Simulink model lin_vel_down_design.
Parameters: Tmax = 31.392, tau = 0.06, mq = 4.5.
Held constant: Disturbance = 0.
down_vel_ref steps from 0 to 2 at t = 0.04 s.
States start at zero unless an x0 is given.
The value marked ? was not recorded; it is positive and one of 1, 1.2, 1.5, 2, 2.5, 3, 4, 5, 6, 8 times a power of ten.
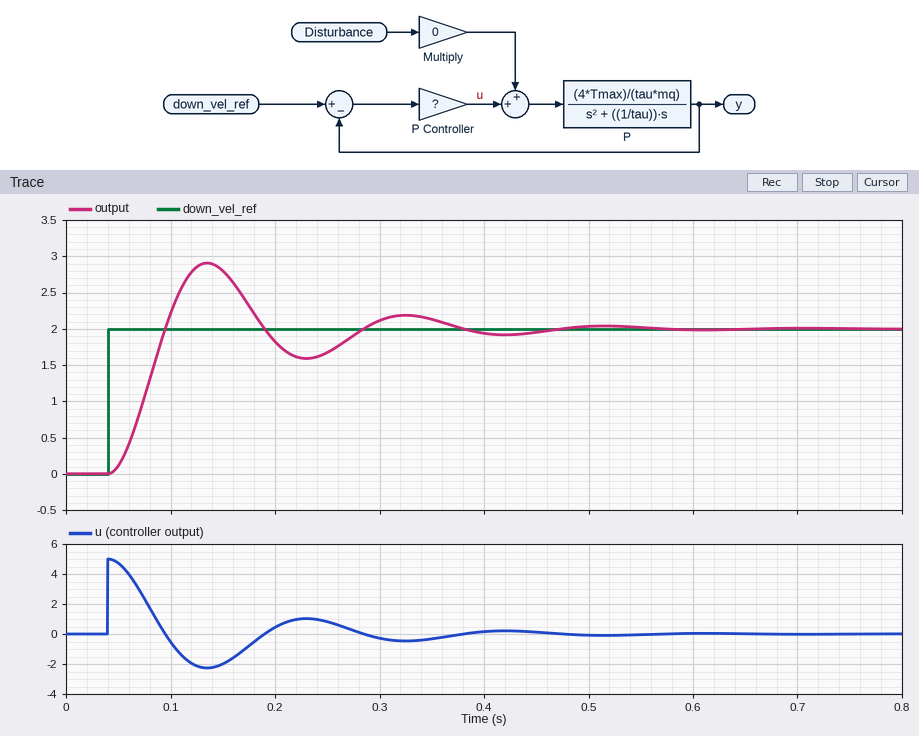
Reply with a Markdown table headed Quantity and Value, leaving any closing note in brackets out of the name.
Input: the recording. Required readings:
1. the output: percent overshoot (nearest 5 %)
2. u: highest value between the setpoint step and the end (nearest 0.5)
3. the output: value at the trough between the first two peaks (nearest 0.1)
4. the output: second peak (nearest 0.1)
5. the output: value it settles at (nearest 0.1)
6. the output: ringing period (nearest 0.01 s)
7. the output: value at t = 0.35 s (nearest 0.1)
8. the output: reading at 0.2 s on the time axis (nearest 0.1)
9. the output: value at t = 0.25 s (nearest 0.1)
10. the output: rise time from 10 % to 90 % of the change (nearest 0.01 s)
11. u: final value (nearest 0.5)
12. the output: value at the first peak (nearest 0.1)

| Quantity | Value |
|---|---|
| the output: percent overshoot | 45 % |
| u: highest value between the setpoint step and the end | 5.0 |
| the output: value at the trough between the first two peaks | 1.6 |
| the output: second peak | 2.2 |
| the output: value it settles at | 2.0 |
| the output: ringing period | 0.19 s |
| the output: value at t = 0.35 s | 2.1 |
| the output: reading at 0.2 s on the time axis | 1.8 |
| the output: value at t = 0.25 s | 1.7 |
| the output: rise time from 10 % to 90 % of the change | 0.04 s |
| u: final value | 0.0 |
| the output: value at the first peak | 2.9 |
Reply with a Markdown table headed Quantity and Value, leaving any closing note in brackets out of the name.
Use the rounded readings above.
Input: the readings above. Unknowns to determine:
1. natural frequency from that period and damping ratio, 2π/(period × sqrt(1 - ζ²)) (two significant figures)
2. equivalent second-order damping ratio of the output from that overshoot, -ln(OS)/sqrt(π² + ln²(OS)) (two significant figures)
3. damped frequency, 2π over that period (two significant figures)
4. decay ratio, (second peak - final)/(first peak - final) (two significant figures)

| Quantity | Value |
|---|---|
| natural frequency from that period and damping ratio, 2π/(period × sqrt(1 - ζ²)) | 34 rad/s |
| equivalent second-order damping ratio of the output from that overshoot, -ln(OS)/sqrt(π² + ln²(OS)) | 0.25 |
| damped frequency, 2π over that period | 33 rad/s |
| decay ratio, (second peak - final)/(first peak - final) | 0.22 |
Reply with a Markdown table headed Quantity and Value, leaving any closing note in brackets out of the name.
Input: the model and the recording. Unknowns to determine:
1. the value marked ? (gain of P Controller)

| Quantity | Value |
|---|---|
| the value marked ? | 2.5 |
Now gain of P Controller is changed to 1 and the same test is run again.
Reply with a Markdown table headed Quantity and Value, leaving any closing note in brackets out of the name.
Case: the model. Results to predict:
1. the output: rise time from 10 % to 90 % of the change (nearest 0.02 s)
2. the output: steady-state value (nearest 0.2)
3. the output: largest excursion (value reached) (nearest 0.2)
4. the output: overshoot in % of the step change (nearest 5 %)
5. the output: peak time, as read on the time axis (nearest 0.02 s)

| Quantity | Value |
|---|---|
| the output: rise time from 10 % to 90 % of the change | 0.06 s |
| the output: steady-state value | 2.0 |
| the output: largest excursion (value reached) | 2.6 |
| the output: overshoot in % of the step change | 25 % |
| the output: peak time, as read on the time axis | 0.20 s |
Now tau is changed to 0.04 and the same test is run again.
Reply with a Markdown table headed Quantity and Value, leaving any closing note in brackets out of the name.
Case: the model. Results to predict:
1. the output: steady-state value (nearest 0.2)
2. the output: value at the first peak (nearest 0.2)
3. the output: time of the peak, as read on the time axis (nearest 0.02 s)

| Quantity | Value |
|---|---|
| the output: steady-state value | 2.0 |
| the output: value at the first peak | 2.8 |
| the output: time of the peak, as read on the time axis | 0.12 s |
